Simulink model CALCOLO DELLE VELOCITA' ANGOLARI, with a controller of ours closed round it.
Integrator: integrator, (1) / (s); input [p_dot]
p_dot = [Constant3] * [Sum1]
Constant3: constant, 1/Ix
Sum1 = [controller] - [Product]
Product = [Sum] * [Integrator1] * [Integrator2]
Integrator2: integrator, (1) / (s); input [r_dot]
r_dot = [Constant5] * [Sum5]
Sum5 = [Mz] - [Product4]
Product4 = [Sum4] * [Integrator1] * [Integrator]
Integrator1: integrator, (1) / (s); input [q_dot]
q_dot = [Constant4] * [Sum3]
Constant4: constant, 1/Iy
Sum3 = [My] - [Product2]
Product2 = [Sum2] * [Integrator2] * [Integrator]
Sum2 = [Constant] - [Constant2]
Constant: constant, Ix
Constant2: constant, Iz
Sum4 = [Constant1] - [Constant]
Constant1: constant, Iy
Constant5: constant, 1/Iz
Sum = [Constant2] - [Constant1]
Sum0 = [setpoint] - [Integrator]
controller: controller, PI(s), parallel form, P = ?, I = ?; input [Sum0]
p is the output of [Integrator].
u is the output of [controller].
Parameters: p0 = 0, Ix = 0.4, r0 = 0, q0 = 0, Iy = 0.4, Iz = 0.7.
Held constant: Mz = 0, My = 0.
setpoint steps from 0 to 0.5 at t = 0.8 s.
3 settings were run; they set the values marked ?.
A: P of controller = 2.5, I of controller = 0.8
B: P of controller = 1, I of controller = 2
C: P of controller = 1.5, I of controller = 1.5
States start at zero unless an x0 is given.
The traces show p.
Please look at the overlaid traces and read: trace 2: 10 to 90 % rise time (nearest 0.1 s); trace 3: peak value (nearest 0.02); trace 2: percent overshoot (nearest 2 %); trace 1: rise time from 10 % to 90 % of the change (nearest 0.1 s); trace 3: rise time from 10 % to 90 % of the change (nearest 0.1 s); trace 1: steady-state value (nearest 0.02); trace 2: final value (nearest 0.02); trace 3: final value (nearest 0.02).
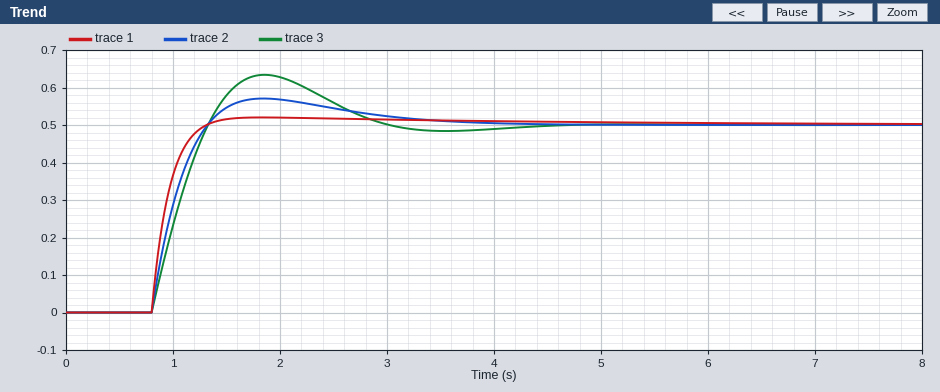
0.4 s
0.64
14 %
0.3 s
0.4 s
0.50
0.50
0.50
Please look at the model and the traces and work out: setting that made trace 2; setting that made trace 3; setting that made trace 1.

C
B
A
